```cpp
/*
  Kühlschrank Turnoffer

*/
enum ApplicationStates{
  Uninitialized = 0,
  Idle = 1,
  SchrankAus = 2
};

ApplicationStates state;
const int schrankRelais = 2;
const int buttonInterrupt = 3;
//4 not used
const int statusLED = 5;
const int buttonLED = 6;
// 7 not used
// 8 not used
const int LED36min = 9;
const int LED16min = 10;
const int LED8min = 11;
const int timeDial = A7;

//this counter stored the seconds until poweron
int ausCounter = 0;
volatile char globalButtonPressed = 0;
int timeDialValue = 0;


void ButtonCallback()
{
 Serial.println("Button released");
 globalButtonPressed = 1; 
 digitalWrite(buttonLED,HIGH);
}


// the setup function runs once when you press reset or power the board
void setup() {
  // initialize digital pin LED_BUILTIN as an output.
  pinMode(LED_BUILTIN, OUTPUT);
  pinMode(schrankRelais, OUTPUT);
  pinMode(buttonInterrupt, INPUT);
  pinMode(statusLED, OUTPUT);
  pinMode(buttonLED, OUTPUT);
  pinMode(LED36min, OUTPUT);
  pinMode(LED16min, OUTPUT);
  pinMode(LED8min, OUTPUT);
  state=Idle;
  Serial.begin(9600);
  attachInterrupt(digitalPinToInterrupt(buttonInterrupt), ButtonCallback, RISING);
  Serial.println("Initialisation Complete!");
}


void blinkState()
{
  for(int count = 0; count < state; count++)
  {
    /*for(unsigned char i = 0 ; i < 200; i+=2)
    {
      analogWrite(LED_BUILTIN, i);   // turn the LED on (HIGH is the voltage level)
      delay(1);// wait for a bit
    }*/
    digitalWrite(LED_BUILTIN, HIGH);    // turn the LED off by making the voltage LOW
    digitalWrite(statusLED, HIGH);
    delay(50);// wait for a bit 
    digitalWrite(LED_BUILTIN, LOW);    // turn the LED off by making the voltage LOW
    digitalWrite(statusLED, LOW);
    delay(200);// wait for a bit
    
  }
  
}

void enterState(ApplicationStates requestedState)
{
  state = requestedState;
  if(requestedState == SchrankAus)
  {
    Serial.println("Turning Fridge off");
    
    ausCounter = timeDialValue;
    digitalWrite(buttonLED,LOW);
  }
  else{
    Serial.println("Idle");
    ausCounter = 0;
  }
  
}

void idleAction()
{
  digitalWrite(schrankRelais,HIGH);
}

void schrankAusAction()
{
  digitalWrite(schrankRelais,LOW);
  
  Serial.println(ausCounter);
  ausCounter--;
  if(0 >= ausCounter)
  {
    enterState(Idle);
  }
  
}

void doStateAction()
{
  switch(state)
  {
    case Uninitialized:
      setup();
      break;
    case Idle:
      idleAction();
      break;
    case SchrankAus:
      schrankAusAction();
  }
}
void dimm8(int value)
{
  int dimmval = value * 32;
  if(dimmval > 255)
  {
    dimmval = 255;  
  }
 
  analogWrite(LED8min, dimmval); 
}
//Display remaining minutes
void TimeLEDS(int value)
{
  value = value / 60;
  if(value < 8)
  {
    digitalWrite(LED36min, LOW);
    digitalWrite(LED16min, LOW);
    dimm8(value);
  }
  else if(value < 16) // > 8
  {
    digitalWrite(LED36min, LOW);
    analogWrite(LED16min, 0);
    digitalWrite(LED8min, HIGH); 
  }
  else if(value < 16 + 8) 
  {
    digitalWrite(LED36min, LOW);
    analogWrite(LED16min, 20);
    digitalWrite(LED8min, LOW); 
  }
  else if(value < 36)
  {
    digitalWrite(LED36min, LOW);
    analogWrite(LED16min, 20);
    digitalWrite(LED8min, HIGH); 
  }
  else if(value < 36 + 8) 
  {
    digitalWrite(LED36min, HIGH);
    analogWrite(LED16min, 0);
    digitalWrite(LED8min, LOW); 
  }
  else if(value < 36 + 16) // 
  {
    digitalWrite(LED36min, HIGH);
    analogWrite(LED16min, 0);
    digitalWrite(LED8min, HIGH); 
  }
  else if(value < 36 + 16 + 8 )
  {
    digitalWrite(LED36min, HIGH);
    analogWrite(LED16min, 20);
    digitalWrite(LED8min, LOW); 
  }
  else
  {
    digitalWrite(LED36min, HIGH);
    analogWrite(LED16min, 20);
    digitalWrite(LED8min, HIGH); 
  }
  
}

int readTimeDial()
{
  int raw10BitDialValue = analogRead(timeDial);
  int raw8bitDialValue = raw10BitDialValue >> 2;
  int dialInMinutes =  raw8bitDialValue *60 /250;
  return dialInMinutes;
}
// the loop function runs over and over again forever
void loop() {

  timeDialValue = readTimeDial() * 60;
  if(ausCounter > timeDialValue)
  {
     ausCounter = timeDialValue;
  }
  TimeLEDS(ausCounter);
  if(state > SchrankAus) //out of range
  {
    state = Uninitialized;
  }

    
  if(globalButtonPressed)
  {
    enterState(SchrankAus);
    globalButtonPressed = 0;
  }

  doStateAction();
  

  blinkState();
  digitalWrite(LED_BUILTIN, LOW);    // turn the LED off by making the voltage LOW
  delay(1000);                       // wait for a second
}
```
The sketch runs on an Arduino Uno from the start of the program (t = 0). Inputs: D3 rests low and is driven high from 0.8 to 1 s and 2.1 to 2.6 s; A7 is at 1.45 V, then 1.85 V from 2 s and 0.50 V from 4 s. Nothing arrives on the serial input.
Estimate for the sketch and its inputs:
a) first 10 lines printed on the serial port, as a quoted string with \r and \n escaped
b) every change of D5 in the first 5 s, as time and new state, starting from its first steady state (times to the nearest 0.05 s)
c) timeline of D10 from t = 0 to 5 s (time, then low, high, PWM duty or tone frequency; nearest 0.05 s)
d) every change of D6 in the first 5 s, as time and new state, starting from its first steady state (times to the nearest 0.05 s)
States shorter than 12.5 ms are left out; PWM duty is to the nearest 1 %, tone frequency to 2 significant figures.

"Initialisation Complete!\r\nButton released\r\nTurning Fridge off\r\n1020\r\nButton released\r\nTurning Fridge off\r\n1320\r\n360\r\n359\r\n358\r\n"
0 s high; 0.05 s low; 1.25 s high; 1.3 s low; 1.5 s high; 1.55 s low; 2.75 s high; 2.8 s low; 3 s high; 3.05 s low; 4.25 s high; 4.3 s low; 4.5 s high; 4.55 s low
0 s low; 2.75 s PWM 8 %; 4.25 s low
0 s low; 0.8 s high; 1.25 s low; 2.1 s high; 2.75 s low
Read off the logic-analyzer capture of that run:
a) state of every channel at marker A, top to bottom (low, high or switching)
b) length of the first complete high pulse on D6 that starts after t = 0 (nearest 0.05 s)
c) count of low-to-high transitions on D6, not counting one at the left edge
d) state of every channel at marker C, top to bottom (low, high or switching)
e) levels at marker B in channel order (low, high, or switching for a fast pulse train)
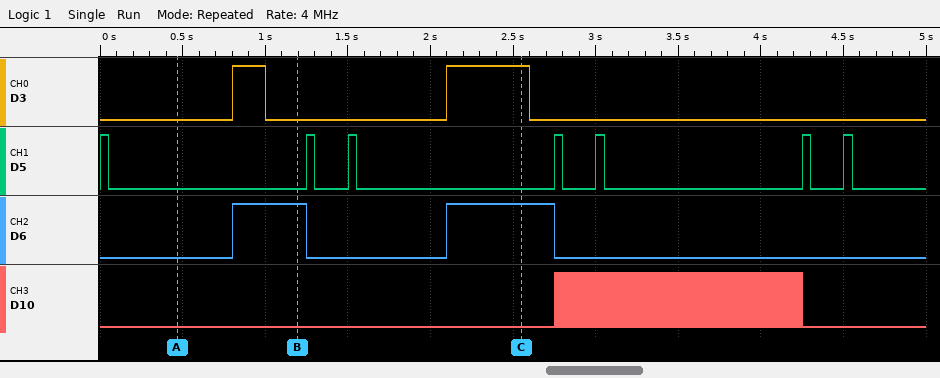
D3 low, D5 low, D6 low, D10 low
0.45 s
2
D3 high, D5 low, D6 high, D10 low
D3 low, D5 low, D6 high, D10 low
